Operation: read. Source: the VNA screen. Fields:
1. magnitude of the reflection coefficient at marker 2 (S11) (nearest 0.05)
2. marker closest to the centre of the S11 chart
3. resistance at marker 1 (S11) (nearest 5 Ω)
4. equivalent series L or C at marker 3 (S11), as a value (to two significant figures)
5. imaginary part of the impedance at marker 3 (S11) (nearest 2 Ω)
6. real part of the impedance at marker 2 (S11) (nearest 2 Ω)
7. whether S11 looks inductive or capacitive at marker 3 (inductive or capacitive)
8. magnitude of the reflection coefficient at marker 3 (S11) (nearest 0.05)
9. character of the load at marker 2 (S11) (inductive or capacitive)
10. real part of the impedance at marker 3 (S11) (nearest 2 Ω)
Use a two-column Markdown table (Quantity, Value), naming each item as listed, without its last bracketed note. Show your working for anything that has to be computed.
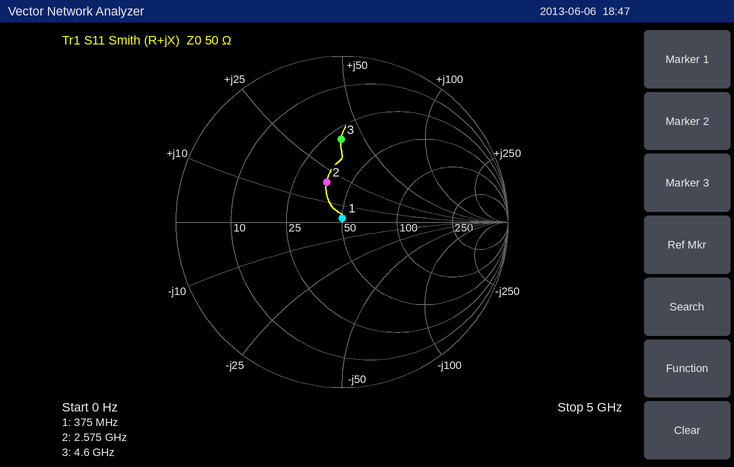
| Quantity | Value |
|---|---|
| magnitude of the reflection coefficient at marker 2 (S11) | 0.25 |
| marker closest to the centre of the S11 chart | marker 1 |
| resistance at marker 1 (S11) | 50 Ω |
| equivalent series L or C at marker 3 (S11), as a value | L = 40 Ω/(2π × 4.6 GHz) ≈ 1.4 nH |
| imaginary part of the impedance at marker 3 (S11) | +40 Ω |
| real part of the impedance at marker 2 (S11) | 38 Ω |
| whether S11 looks inductive or capacitive at marker 3 | inductive |
| magnitude of the reflection coefficient at marker 3 (S11) | 0.50 |
| character of the load at marker 2 (S11) | inductive |
| real part of the impedance at marker 3 (S11) | 30 Ω |
